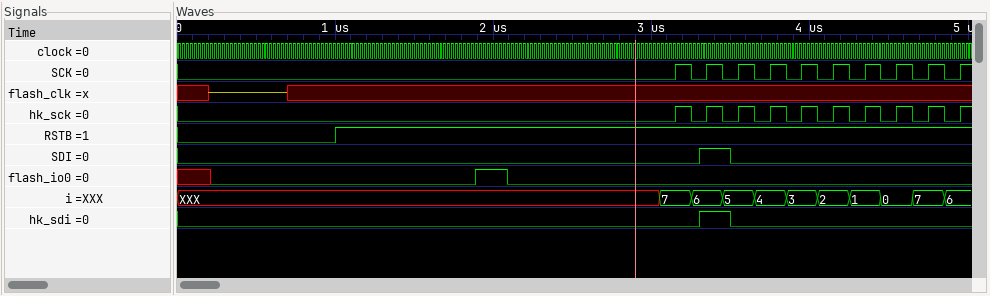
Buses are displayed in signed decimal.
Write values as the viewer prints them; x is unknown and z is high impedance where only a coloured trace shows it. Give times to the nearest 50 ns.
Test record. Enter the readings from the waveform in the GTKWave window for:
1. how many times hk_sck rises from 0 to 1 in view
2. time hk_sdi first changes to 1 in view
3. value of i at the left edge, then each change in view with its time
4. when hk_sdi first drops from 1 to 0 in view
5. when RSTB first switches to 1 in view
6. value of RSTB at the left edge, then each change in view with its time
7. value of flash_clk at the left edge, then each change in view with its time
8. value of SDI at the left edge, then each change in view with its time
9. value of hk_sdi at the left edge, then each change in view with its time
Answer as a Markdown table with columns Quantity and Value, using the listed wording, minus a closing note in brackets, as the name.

| Quantity | Value |
|---|---|
| how many times hk_sck rises from 0 to 1 in view | 10 |
| time hk_sdi first changes to 1 in view | 3300 ns |
| value of i at the left edge, then each change in view with its time | XXX, 7 at 3050 ns, 6 at 3250 ns, 5 at 3450 ns, 4 at 3650 ns, 3 at 3850 ns, 2 at 4050 ns, 1 at 4250 ns, 0 at 4450 ns, 7 at 4650 ns, 6 at 4850 ns |
| when hk_sdi first drops from 1 to 0 in view | 3500 ns |
| when RSTB first switches to 1 in view | 1000 ns |
| value of RSTB at the left edge, then each change in view with its time | 0, 1 at 1000 ns |
| value of flash_clk at the left edge, then each change in view with its time | x, z at 200 ns, x at 700 ns |
| value of SDI at the left edge, then each change in view with its time | 0, 1 at 3300 ns, 0 at 3500 ns |
| value of hk_sdi at the left edge, then each change in view with its time | 0, 1 at 3300 ns, 0 at 3500 ns |
